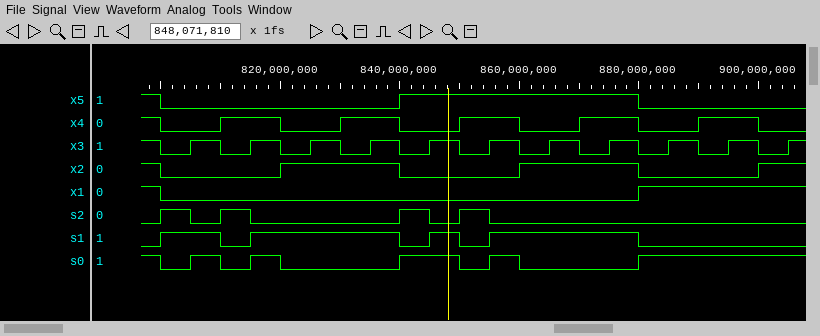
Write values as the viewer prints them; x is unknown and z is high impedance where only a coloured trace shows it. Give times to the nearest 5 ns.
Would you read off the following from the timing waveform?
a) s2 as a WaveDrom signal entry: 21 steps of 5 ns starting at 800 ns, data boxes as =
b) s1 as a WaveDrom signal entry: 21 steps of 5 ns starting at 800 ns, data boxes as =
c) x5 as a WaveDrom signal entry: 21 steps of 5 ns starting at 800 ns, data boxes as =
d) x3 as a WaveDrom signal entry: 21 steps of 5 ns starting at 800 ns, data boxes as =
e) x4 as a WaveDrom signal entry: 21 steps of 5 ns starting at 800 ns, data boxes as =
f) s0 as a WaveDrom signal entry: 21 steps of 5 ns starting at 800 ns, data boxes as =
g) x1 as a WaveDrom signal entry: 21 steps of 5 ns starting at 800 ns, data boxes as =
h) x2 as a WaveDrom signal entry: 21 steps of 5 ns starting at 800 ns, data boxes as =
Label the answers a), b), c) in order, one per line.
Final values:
a) {name: 's2', wave: '1010....1010.........'}
b) {name: 's1', wave: '1.01....0101....0....'}
c) {name: 'x5', wave: '0.......1.......0....'}
d) {name: 'x3', wave: '010101010101010101010'}
e) {name: 'x4', wave: '0.1.0.1.0.1.0.1.0.1.0'}
f) {name: 's0', wave: '01010...1.010...1....'}
g) {name: 'x1', wave: '0...............1....'}
h) {name: 'x2', wave: '0...1...0...1...0...1'}
